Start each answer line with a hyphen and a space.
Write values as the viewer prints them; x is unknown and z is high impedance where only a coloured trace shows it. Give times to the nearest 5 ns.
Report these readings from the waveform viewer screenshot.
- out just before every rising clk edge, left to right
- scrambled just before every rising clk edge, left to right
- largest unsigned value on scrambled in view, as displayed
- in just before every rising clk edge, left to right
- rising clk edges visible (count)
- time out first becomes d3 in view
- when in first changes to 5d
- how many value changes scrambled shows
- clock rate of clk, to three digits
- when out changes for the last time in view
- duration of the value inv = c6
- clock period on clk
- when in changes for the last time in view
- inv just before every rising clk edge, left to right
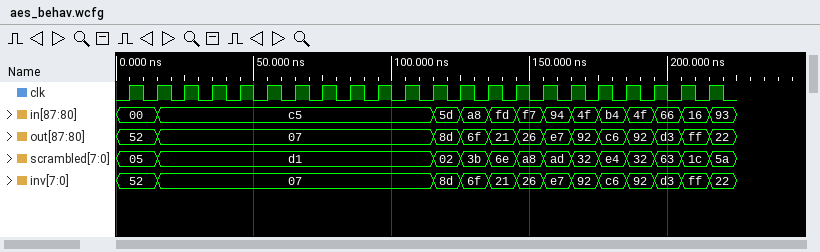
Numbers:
- 52, 52, 07, 07, 07, 07, 07, 07, 07, 07, 07, 07, 8d, 6f, 21, 26, e7, 92, c6, 92, d3, ff
- 05, 05, d1, d1, d1, d1, d1, d1, d1, d1, d1, d1, 02, 3b, 6e, a8, ad, 32, e4, 32, 63, 1c
- e4
- 00, 00, c5, c5, c5, c5, c5, c5, c5, c5, c5, c5, 5d, a8, fd, f7, 94, 4f, b4, 4f, 66, 16
- 22
- 195 ns
- 115 ns
- 12
- 100 MHz
- 215 ns
- 10 ns
- 10 ns
- 215 ns
- 52, 52, 07, 07, 07, 07, 07, 07, 07, 07, 07, 07, 8d, 6f, 21, 26, e7, 92, c6, 92, d3, ff
